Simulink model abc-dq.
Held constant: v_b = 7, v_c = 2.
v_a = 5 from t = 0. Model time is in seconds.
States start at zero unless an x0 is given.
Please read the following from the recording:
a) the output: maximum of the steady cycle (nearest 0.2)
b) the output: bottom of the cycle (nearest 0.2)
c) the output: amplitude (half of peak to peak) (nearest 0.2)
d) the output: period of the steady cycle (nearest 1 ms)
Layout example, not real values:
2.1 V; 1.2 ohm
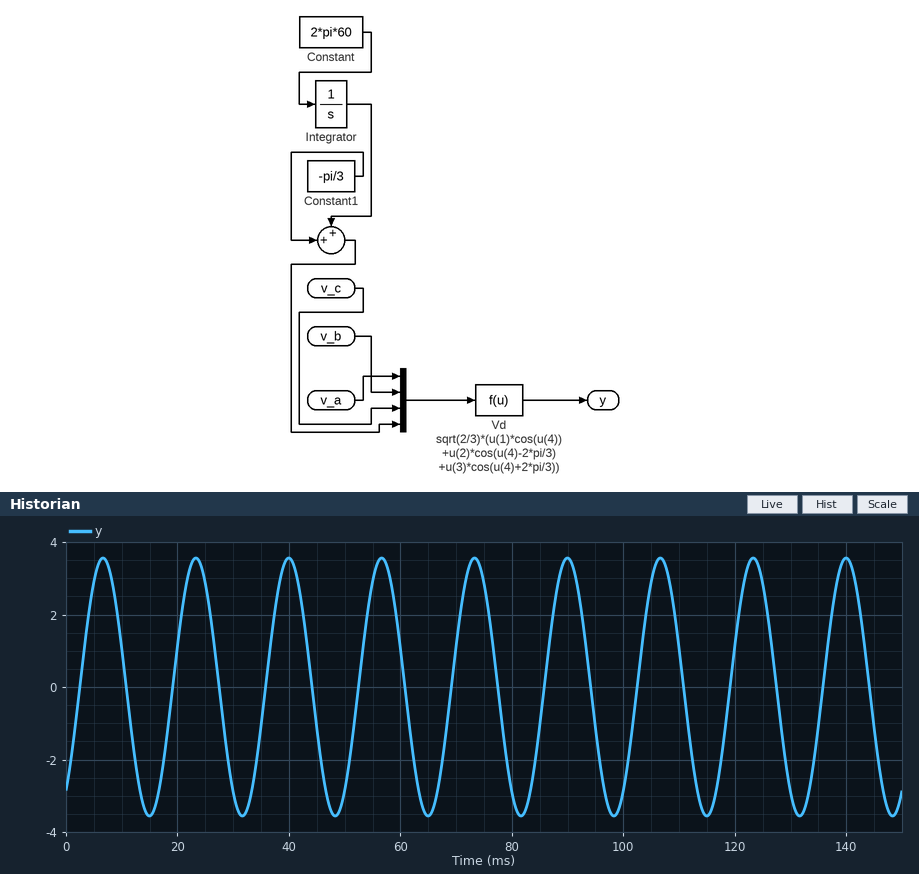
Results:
3.6; -3.6; 3.6; 17 ms
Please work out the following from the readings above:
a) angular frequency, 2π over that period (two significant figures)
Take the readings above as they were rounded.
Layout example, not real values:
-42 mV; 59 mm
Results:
0.37 rad/ms
